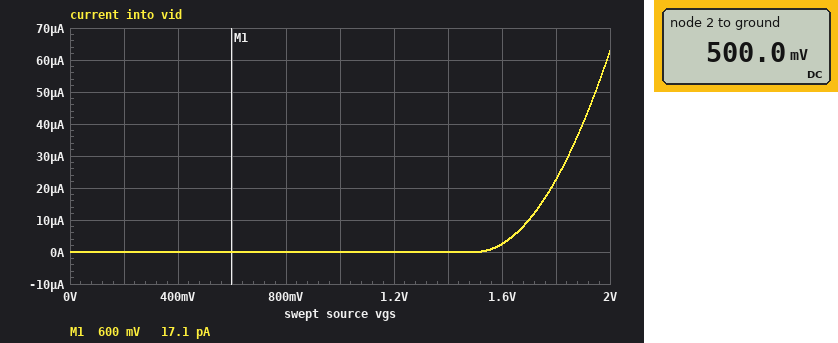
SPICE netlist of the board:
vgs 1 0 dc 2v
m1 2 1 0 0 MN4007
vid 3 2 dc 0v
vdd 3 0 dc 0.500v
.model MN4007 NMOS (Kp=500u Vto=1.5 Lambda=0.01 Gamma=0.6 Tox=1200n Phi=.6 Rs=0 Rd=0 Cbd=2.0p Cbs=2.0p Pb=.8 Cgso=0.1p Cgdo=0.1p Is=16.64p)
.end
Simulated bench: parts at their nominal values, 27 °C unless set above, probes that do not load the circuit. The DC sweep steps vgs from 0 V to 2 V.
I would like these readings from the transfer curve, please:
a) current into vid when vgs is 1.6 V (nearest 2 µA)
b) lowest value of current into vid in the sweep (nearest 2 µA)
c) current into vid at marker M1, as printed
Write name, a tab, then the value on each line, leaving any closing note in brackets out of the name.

current into vid when vgs is 1.6 V	2 µA
lowest value of current into vid in the sweep	0 A
current into vid at marker M1, as printed	17.1 pA
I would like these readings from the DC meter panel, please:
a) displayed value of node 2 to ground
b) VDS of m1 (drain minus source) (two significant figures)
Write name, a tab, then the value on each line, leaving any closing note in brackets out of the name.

displayed value of node 2 to ground	500.0 mV
VDS of m1 (drain minus source)	500 mV
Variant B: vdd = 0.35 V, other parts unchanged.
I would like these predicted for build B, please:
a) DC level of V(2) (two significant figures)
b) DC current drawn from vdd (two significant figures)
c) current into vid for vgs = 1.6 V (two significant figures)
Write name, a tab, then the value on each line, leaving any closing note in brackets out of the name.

DC level of V(2)	350 mV
DC current drawn from vdd	57 µA
current into vid for vgs = 1.6 V	2.5 µA
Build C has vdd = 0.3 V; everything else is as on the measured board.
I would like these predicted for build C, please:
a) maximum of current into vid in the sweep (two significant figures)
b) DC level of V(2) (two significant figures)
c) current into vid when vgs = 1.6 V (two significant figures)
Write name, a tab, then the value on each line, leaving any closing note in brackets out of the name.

maximum of current into vid in the sweep	53 µA
DC level of V(2)	300 mV
current into vid when vgs = 1.6 V	2.5 µA
